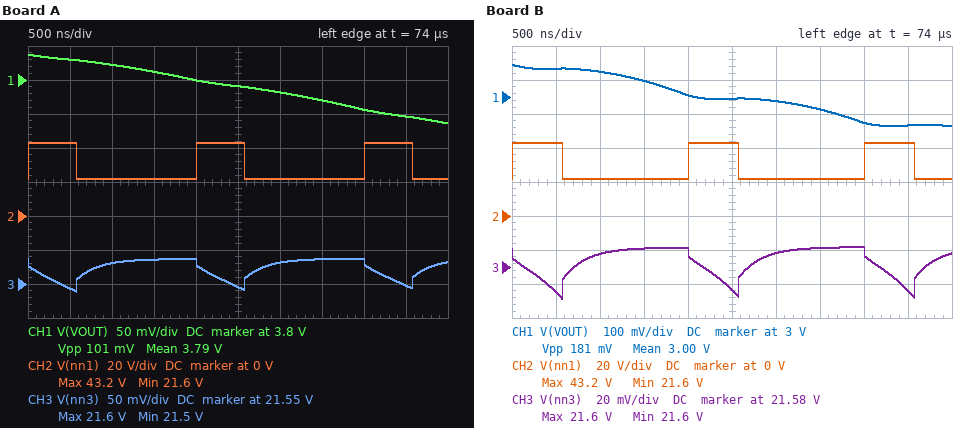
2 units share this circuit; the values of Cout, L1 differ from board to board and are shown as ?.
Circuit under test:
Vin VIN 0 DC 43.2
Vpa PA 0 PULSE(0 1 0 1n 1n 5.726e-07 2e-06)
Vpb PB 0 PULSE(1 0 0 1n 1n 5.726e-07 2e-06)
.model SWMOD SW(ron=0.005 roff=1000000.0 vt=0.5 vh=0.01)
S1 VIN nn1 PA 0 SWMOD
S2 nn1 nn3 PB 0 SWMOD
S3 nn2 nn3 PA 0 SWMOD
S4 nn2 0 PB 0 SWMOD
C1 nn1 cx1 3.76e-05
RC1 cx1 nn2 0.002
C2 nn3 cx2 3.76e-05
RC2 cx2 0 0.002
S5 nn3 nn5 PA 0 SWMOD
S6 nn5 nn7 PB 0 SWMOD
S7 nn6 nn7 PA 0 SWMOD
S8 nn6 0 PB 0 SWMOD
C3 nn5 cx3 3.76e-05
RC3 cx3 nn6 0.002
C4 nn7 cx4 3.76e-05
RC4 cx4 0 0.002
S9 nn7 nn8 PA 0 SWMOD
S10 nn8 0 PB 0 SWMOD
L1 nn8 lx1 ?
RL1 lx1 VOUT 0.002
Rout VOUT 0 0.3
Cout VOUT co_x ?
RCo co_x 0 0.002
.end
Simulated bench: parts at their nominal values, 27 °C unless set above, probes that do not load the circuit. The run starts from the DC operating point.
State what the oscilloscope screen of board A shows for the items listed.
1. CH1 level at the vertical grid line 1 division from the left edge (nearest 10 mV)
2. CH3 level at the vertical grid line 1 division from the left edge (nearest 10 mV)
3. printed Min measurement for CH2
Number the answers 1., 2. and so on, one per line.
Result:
1. 3.83 V
2. 21.54 V
3. 21.6 V
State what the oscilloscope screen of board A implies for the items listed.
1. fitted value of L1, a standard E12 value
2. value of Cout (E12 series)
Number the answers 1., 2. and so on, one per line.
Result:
1. 3.9 µH
2. 100 µF
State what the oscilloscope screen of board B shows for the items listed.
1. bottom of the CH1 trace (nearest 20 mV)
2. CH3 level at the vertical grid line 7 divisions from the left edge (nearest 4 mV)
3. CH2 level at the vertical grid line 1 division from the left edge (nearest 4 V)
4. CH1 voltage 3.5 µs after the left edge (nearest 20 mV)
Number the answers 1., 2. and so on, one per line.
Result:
1. 2.92 V
2. 21.592 V
3. 44 V
4. 2.96 V
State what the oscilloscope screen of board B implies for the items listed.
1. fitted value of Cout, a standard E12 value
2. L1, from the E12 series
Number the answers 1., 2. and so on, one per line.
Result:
1. 82 µF
2. 560 nH
